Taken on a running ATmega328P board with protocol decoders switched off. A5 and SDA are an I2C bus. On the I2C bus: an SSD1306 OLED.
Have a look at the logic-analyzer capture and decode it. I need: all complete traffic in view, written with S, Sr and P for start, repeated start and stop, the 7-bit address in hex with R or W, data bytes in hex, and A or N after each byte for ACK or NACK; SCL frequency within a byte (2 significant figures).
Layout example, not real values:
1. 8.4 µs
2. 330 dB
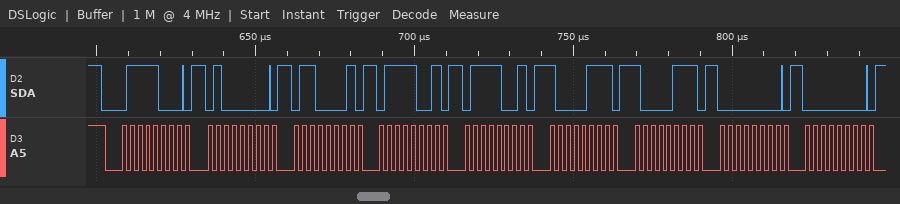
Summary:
1. S 3CW A 40 A 61 A 79 A 79 A 87 A 87 A 00 A 00 A
2. 400 kHz
